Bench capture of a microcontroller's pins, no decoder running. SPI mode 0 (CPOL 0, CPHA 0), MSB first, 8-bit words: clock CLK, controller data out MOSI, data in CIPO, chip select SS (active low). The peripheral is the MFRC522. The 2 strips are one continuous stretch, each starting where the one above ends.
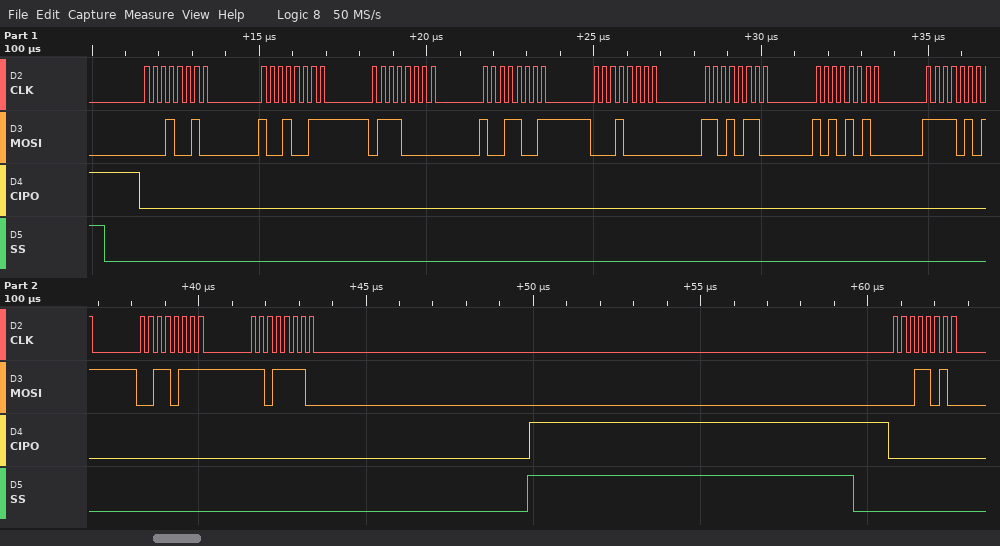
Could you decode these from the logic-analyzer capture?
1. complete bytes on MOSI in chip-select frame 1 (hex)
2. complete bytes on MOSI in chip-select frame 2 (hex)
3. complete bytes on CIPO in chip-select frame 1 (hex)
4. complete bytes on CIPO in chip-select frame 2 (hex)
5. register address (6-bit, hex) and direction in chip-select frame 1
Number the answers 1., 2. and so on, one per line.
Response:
1. 0x12 0x93 0x70 0x99 0x10 0xD6 0xAA 0xF5 0x37 0xDE
2. 0x1A
3. 0x00 0x00 0x00 0x00 0x00 0x00 0x00 0x00 0x00 0x00
4. 0x00
5. 0x09 write
